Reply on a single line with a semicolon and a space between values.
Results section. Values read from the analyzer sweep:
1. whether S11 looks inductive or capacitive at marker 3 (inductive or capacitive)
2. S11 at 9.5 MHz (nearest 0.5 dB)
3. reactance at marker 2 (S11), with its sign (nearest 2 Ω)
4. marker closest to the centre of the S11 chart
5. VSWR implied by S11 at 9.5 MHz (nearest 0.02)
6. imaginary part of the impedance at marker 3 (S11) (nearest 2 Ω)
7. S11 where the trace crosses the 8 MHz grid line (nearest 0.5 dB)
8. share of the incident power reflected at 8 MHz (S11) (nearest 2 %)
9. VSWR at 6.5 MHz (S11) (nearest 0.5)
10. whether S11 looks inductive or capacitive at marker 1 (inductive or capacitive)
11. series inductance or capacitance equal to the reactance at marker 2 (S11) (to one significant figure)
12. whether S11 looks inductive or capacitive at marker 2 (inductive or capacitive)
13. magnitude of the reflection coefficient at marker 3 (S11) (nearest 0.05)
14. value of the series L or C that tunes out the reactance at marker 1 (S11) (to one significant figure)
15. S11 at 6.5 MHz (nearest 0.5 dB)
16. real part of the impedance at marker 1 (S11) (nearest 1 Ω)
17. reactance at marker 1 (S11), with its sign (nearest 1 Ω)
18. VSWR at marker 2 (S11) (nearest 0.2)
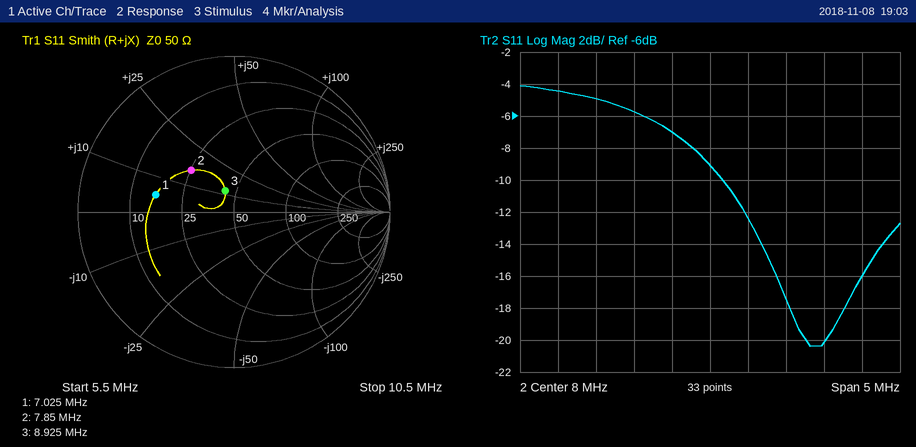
inductive; -20.0 dB; +16 Ω; marker 3; 1.22; +12 Ω; -9.0 dB; 12 %; 3.5; inductive; 300 nH; inductive; 0.15; 5 nF; -5.0 dB; 16 Ω; +5 Ω; 2.2
